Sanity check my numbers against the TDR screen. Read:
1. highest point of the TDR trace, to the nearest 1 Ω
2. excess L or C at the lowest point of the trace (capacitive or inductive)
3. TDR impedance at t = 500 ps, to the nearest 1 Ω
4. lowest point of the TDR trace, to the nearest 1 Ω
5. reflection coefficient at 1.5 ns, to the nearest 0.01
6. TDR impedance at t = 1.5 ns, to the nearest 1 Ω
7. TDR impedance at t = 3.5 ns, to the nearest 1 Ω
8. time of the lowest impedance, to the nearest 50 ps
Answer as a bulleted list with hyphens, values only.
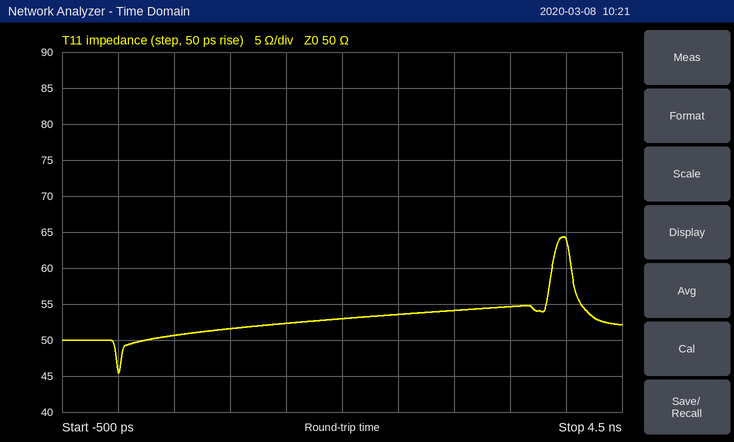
- 64 Ω
- capacitive
- 51 Ω
- 45 Ω
- +0.02
- 52 Ω
- 55 Ω
- 0 ps
